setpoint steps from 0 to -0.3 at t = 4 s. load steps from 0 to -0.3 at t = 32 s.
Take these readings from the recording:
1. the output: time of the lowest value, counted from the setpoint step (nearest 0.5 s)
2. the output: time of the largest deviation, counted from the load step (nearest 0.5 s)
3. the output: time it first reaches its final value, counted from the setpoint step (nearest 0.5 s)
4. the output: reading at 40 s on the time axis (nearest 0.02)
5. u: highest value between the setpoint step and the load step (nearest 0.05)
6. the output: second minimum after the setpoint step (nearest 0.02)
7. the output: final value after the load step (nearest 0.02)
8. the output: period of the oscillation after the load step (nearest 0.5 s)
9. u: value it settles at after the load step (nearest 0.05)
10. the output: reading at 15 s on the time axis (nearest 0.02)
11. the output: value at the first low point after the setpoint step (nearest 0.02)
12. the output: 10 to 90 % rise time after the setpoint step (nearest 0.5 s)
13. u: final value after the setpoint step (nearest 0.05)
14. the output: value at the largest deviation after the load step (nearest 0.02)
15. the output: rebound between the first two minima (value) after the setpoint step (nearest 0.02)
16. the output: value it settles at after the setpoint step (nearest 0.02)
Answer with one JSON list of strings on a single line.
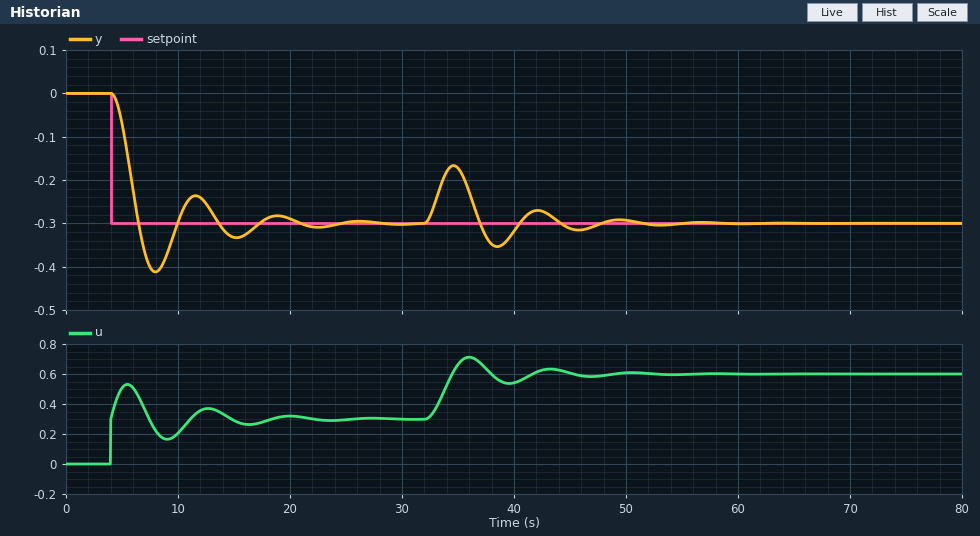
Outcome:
["4.0 s", "2.5 s", "2.5 s", "-0.32", "0.55", "-0.34", "-0.30", "7.5 s", "0.60", "-0.34", "-0.42", "1.5 s", "0.30", "-0.16", "-0.24", "-0.30"]
